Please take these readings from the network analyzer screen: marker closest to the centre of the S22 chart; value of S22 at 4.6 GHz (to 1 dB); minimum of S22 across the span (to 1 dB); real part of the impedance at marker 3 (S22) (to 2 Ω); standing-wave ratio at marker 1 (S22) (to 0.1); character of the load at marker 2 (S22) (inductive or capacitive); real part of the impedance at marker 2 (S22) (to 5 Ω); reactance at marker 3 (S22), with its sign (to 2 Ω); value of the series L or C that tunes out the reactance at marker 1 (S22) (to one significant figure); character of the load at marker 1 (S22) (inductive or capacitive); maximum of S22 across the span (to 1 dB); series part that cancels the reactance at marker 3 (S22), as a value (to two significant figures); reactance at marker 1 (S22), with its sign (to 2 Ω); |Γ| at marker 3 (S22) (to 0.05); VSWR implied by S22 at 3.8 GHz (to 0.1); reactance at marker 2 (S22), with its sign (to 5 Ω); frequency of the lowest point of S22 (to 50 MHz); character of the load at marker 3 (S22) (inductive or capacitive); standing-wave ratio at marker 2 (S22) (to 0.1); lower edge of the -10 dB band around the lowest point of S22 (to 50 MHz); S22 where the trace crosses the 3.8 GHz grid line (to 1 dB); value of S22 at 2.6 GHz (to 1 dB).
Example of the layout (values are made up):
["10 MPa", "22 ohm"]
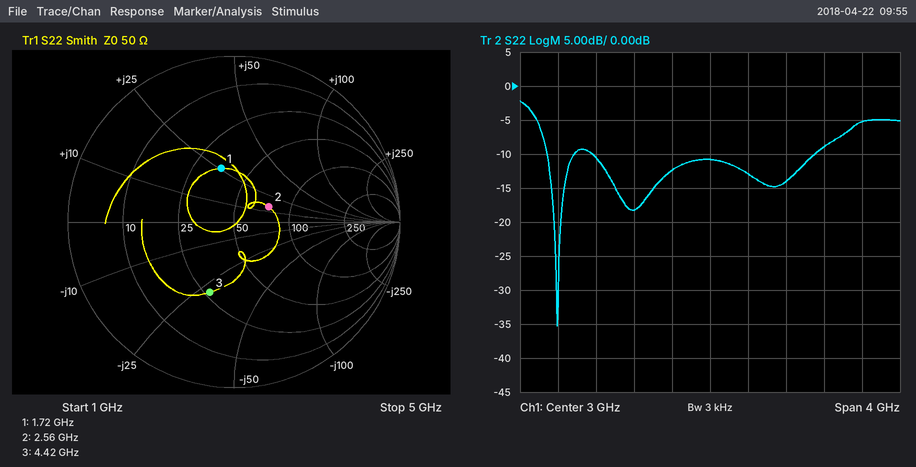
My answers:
["marker 2", "-5 dB", "-35 dB", "26 Ω", "2.0", "inductive", "75 Ω", "-28 Ω", "4 pF", "inductive", "-2 dB", "1.0 nH", "+26 Ω", "0.45", "1.5", "+15 Ω", "1.40 GHz", "capacitive", "1.6", "1.30 GHz", "-14 dB", "-12 dB"]
